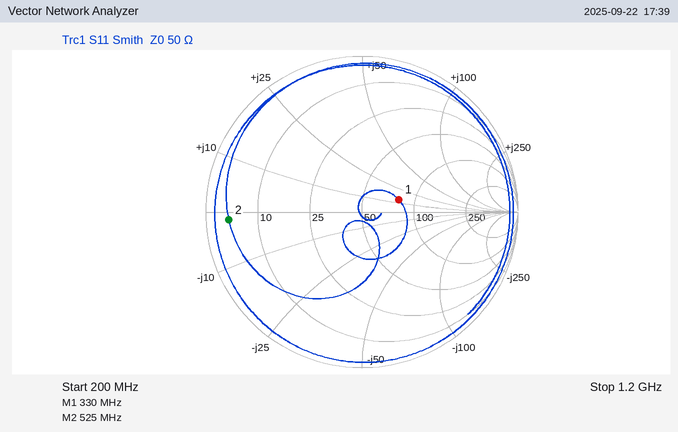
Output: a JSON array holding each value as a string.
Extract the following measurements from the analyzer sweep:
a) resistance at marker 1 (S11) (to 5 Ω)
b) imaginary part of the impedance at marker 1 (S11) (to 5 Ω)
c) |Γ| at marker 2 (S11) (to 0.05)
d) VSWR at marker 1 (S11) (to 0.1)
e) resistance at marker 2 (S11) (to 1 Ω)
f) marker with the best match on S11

["80 Ω", "+15 Ω", "0.85", "1.7", "4 Ω", "marker 1"]
